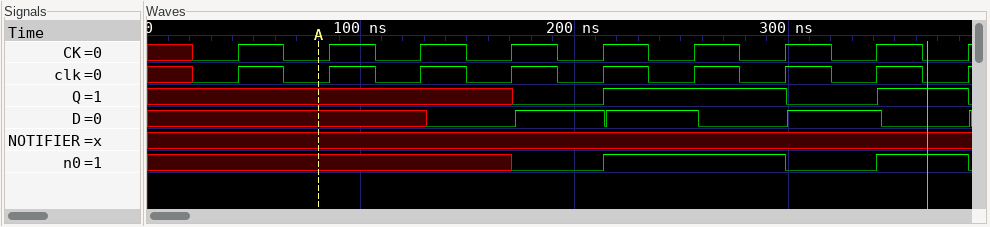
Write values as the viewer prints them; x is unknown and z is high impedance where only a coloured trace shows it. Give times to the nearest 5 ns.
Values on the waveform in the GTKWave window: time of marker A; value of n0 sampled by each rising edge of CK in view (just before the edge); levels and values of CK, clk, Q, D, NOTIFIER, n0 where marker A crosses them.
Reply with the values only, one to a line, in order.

80 ns
x x x x 0 1 1 0 1
CK=0, clk=0, Q=x, D=x, NOTIFIER=x, n0=x
